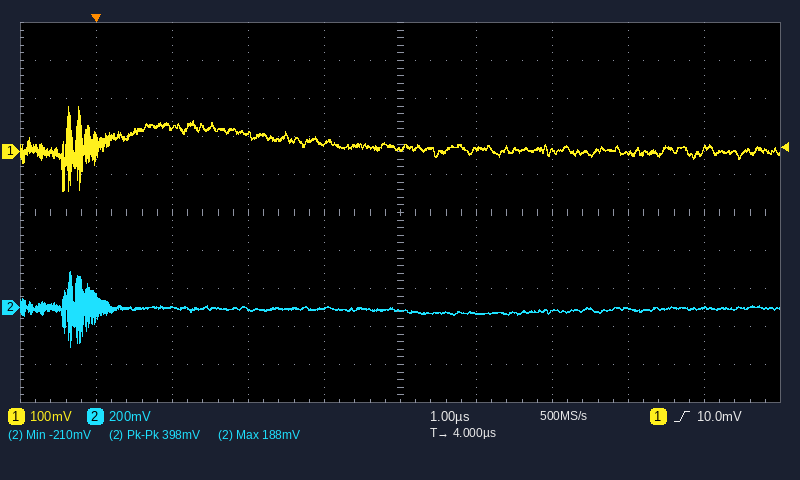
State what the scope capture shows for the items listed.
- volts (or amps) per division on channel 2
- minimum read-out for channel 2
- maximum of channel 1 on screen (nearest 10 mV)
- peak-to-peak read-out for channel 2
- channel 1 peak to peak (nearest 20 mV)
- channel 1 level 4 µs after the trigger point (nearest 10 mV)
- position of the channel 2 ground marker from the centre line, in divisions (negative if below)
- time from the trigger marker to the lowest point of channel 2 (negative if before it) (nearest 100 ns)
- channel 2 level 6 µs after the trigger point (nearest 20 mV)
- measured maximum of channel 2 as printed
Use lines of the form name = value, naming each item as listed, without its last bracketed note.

volts (or amps) per division on channel 2 = 200 mV
minimum read-out for channel 2 = -210 mV
maximum of channel 1 on screen = 120 mV
peak-to-peak read-out for channel 2 = 398 mV
channel 1 peak to peak = 220 mV
channel 1 level 4 µs after the trigger point = 10 mV
position of the channel 2 ground marker from the centre line, in divisions = -2.5 div
time from the trigger marker to the lowest point of channel 2 (negative if before it) = -300 ns
channel 2 level 6 µs after the trigger point = -20 mV
measured maximum of channel 2 as printed = 188 mV
